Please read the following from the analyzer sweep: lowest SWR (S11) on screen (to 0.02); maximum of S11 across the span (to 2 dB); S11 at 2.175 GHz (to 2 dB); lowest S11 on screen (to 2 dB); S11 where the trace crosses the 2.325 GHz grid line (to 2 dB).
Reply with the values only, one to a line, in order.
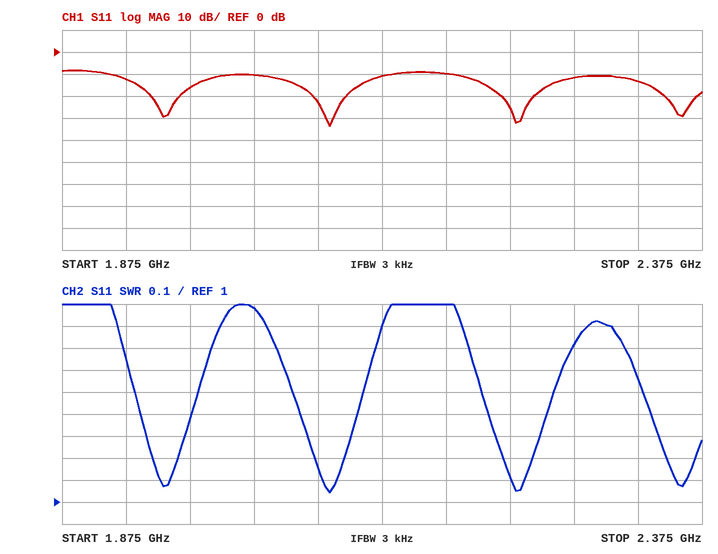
1.04
-8 dB
-10 dB
-34 dB
-14 dB
